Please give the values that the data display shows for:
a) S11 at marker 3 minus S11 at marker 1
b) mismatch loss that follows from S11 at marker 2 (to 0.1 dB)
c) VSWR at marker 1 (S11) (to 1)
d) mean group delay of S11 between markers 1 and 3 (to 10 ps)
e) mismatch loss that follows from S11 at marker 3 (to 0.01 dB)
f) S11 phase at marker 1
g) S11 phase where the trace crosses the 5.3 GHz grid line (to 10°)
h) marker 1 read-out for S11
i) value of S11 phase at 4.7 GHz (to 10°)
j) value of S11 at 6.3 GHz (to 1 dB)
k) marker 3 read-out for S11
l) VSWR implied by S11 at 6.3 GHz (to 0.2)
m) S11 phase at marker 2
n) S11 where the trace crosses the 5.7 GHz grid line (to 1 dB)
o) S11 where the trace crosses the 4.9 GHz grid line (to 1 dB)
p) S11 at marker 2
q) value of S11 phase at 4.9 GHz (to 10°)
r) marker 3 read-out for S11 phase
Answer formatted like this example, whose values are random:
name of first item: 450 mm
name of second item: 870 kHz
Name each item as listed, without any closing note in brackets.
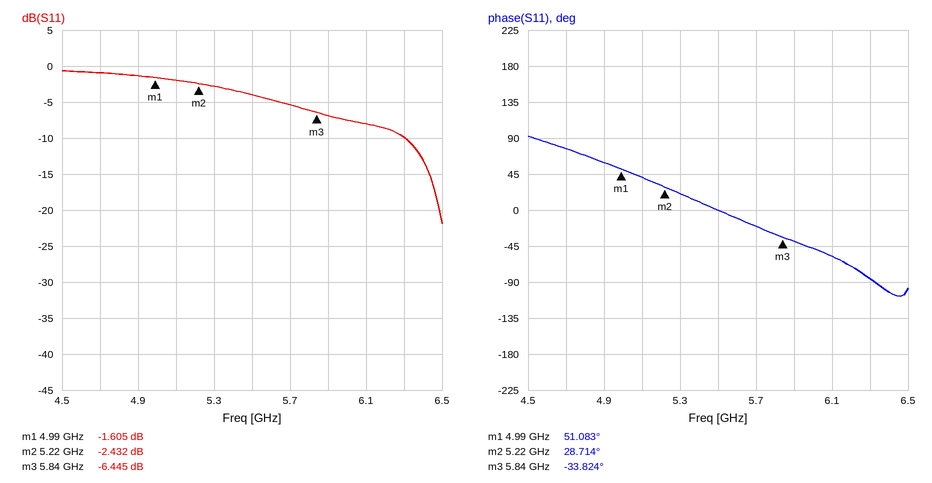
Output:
S11 at marker 3 minus S11 at marker 1: -4.840 dB
mismatch loss that follows from S11 at marker 2: 3.7 dB
VSWR at marker 1 (S11): 11
mean group delay of S11 between markers 1 and 3: 280 ps
mismatch loss that follows from S11 at marker 3: 1.12 dB
S11 phase at marker 1: 51.083°
S11 phase where the trace crosses the 5.3 GHz grid line: 20°
marker 1 read-out for S11: -1.605 dB
value of S11 phase at 4.7 GHz: 80°
value of S11 at 6.3 GHz: -10 dB
marker 3 read-out for S11: -6.445 dB
VSWR implied by S11 at 6.3 GHz: 2.0
S11 phase at marker 2: 28.714°
S11 where the trace crosses the 5.7 GHz grid line: -5 dB
S11 where the trace crosses the 4.9 GHz grid line: -1 dB
S11 at marker 2: -2.432 dB
value of S11 phase at 4.9 GHz: 60°
marker 3 read-out for S11 phase: -33.824°
